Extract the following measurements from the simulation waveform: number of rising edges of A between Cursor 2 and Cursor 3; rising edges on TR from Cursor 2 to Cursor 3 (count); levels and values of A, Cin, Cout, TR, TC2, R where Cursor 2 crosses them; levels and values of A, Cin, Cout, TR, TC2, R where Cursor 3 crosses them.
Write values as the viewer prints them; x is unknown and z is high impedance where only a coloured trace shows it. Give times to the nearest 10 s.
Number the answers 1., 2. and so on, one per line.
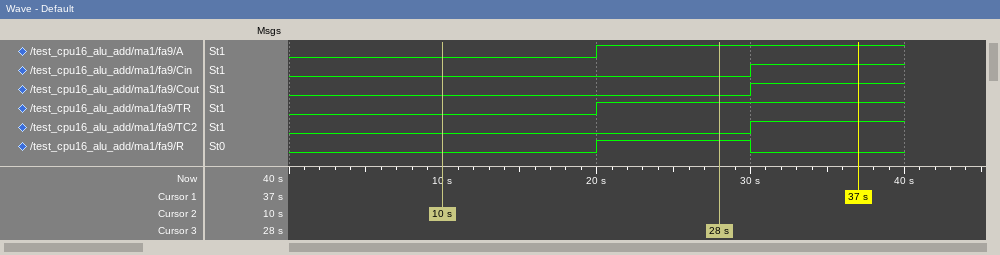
1. 1
2. 1
3. A=0, Cin=0, Cout=0, TR=0, TC2=0, R=0
4. A=1, Cin=0, Cout=0, TR=1, TC2=0, R=1
